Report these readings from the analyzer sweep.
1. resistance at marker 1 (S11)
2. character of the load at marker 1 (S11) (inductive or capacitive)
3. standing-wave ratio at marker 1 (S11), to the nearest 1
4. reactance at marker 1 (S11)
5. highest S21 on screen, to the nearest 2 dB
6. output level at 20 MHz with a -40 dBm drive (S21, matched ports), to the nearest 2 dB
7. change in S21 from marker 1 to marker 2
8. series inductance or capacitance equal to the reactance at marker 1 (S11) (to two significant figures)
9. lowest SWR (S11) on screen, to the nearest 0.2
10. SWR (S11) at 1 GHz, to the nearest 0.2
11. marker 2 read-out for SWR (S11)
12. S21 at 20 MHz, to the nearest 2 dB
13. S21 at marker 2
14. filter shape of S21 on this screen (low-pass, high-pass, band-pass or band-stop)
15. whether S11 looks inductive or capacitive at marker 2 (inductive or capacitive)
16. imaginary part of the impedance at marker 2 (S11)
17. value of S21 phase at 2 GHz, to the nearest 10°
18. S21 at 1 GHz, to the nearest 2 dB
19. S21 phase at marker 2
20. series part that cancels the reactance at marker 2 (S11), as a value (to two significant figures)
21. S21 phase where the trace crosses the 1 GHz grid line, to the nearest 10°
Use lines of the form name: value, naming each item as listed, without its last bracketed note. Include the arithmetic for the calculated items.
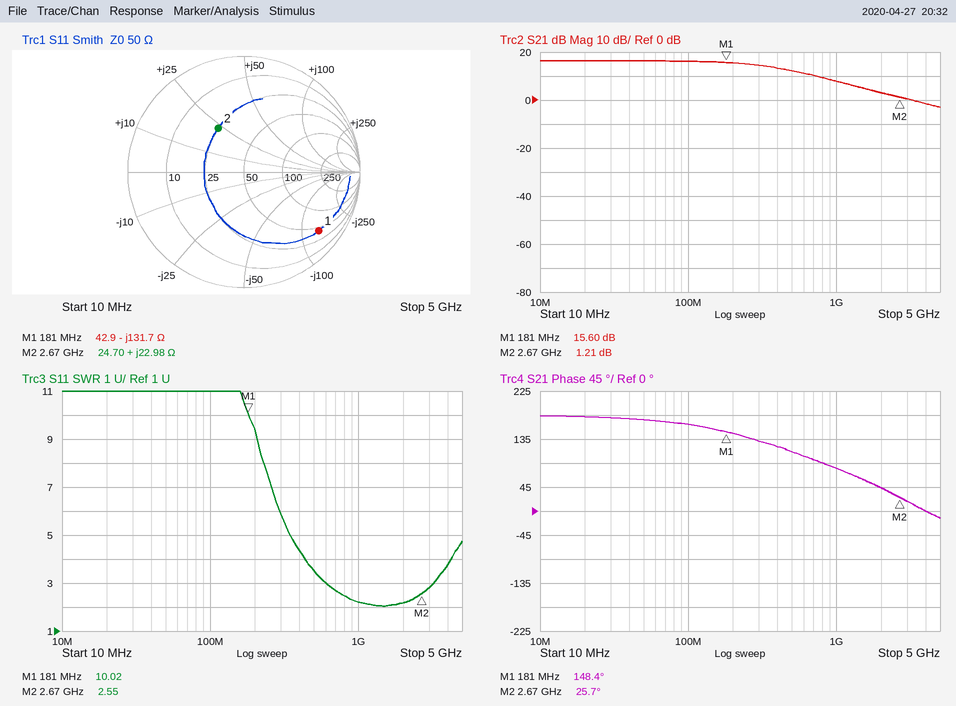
resistance at marker 1: 42.9 Ω
character of the load at marker 1 (S11): capacitive
standing-wave ratio at marker 1 (S11), to the nearest 1: 10
reactance at marker 1: -131.7 Ω
highest S21 on screen, to the nearest 2 dB: 16 dB
output level at 20 MHz with a -40 dBm drive (S21, matched ports), to the nearest 2 dB: -40 dBm + (16 dB) = -24 dBm
change in S21 from marker 1 to marker 2: 1.21 − (15.6) = -14.39 dB
series inductance or capacitance equal to the reactance at marker 1 (S11): C = 1/(2π × 181 MHz × 131.7 Ω) ≈ 6.7 pF
lowest SWR (S11) on screen, to the nearest 0.2: 2.0
SWR (S11) at 1 GHz, to the nearest 0.2: 2.2
marker 2 read-out for SWR: 2.55
S21 at 20 MHz, to the nearest 2 dB: 16 dB
S21 at marker 2: 1.21 dB
filter shape of S21 on this screen: low-pass
whether S11 looks inductive or capacitive at marker 2: inductive
imaginary part of the impedance at marker 2: +22.98 Ω
value of S21 phase at 2 GHz, to the nearest 10°: 40°
S21 at 1 GHz, to the nearest 2 dB: 8 dB
S21 phase at marker 2: 25.7°
series part that cancels the reactance at marker 2 (S11), as a value: C = 1/(2π × 2.67 GHz × 22.98 Ω) ≈ 2.6 pF
S21 phase where the trace crosses the 1 GHz grid line, to the nearest 10°: 80°
